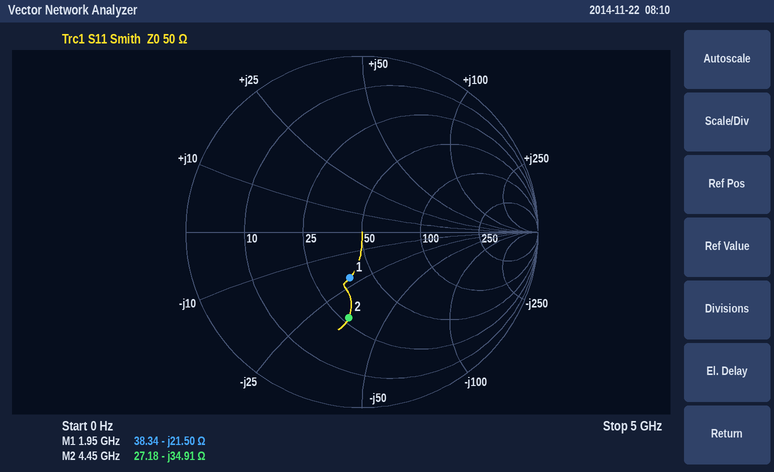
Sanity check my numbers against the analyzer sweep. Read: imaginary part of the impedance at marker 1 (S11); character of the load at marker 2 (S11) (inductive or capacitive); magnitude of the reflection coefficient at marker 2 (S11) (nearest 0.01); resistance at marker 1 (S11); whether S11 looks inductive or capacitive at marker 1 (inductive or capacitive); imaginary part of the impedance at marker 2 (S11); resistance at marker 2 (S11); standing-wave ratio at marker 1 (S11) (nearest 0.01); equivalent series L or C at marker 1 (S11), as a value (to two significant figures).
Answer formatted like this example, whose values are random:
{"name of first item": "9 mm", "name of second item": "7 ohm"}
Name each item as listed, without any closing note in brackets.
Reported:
{"imaginary part of the impedance at marker 1": "-21.50 Ω", "character of the load at marker 2 (S11)": "capacitive", "magnitude of the reflection coefficient at marker 2 (S11)": "0.49", "resistance at marker 1": "38.34 Ω", "whether S11 looks inductive or capacitive at marker 1": "capacitive", "imaginary part of the impedance at marker 2": "-34.91 Ω", "resistance at marker 2": "27.18 Ω", "standing-wave ratio at marker 1 (S11)": "1.74", "equivalent series L or C at marker 1 (S11), as a value": "3.8 pF"}
